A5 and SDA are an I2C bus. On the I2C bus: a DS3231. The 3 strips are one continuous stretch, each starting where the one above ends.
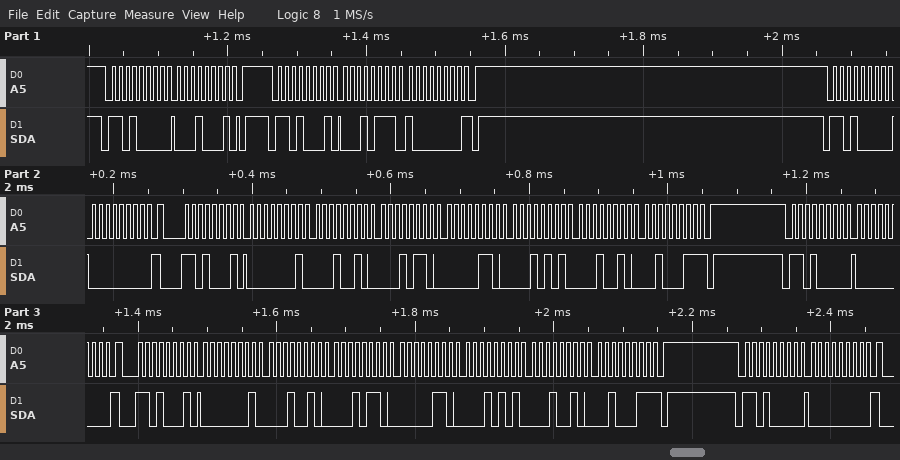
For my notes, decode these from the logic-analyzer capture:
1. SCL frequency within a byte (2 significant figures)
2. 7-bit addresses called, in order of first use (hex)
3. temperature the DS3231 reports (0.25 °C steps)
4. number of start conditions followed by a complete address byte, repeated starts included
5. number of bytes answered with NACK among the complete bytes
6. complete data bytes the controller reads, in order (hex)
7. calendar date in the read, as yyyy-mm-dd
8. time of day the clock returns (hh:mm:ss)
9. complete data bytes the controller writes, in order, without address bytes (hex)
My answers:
100 kHz
0x68
23.50 °C
7
3
17 80 01 12 16 06 15 12 23 01 12 16 06 15 12 23
2023-12-15
16:12:01
11 00 00 00
